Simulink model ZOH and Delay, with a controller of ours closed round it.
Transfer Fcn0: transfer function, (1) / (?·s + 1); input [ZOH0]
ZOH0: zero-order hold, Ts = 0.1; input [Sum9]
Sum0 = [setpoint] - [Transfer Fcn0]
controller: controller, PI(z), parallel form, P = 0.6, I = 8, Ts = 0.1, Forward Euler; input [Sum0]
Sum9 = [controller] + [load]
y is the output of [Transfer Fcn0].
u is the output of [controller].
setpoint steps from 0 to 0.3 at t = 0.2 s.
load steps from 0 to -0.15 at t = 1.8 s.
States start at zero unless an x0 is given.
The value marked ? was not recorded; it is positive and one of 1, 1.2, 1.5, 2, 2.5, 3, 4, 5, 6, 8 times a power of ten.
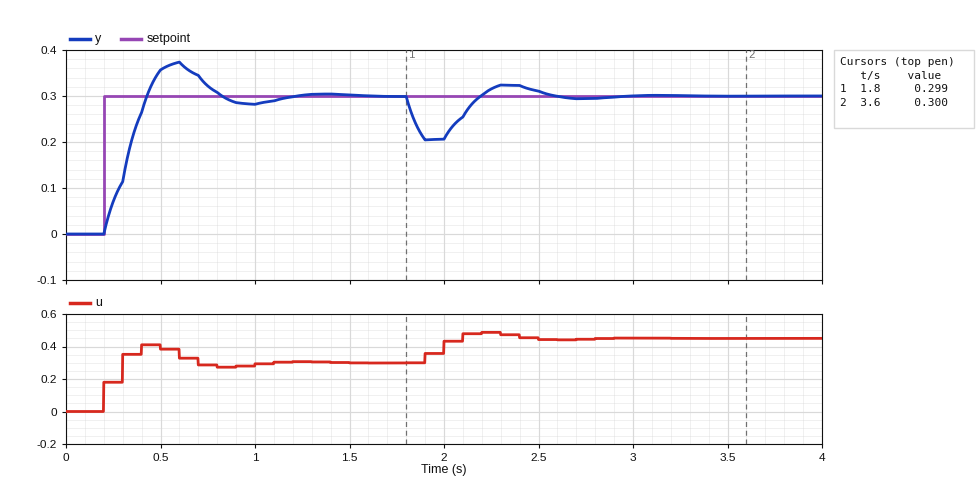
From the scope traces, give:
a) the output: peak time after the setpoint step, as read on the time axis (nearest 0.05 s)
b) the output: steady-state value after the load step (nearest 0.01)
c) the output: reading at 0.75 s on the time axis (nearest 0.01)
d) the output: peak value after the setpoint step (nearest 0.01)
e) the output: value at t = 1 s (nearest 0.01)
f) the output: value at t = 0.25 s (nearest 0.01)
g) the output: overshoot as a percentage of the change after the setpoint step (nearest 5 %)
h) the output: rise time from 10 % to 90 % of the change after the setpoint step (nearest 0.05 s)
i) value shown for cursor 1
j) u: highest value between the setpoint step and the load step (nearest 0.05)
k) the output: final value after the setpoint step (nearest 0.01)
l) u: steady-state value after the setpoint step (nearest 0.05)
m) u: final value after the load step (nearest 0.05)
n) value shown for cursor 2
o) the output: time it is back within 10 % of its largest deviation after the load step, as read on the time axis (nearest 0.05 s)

0.60 s
0.30
0.32
0.37
0.28
0.07
25 %
0.20 s
0.299
0.40
0.30
0.30
0.45
0.300
2.50 s
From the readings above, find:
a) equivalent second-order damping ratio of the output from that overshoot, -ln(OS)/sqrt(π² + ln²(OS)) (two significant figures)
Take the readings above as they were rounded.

0.40
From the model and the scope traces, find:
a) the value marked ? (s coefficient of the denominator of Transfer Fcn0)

0.1
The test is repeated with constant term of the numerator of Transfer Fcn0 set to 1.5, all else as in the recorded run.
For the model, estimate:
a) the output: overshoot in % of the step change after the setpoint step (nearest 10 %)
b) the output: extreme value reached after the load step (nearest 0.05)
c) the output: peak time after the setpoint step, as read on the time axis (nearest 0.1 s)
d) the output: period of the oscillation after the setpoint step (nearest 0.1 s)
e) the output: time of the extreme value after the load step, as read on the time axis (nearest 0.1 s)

40 %
0.15
0.5 s
0.6 s
1.9 s
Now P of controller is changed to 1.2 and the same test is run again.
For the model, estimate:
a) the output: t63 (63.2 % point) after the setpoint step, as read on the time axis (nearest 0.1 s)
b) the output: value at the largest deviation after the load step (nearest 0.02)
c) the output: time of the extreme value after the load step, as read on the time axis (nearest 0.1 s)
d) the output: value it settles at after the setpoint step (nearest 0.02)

0.3 s
0.20
1.9 s
0.30
